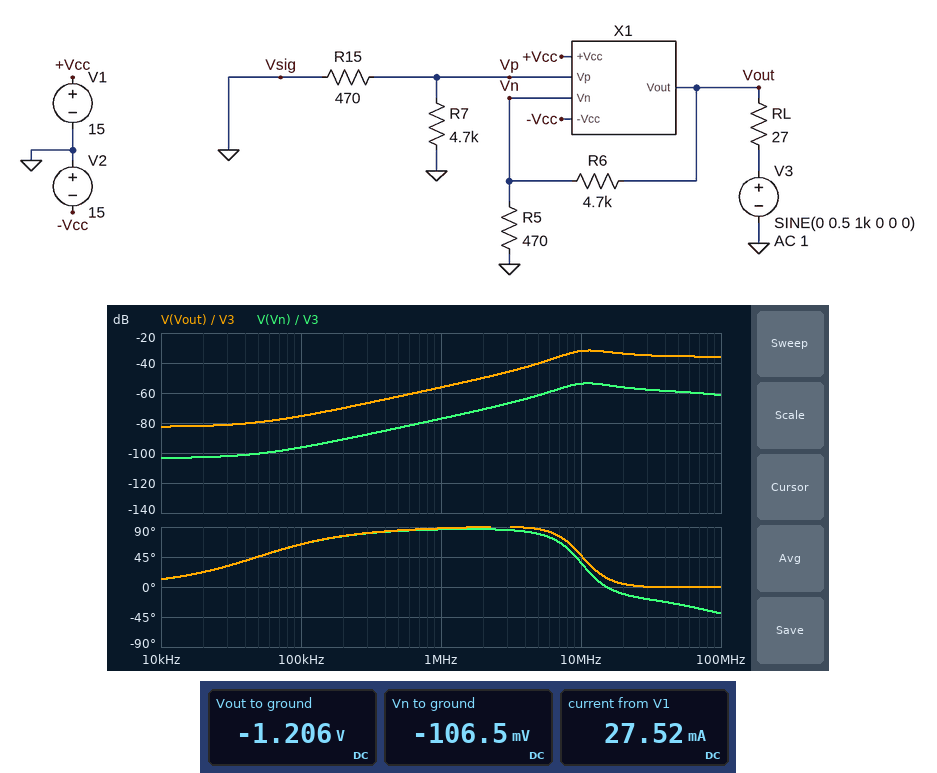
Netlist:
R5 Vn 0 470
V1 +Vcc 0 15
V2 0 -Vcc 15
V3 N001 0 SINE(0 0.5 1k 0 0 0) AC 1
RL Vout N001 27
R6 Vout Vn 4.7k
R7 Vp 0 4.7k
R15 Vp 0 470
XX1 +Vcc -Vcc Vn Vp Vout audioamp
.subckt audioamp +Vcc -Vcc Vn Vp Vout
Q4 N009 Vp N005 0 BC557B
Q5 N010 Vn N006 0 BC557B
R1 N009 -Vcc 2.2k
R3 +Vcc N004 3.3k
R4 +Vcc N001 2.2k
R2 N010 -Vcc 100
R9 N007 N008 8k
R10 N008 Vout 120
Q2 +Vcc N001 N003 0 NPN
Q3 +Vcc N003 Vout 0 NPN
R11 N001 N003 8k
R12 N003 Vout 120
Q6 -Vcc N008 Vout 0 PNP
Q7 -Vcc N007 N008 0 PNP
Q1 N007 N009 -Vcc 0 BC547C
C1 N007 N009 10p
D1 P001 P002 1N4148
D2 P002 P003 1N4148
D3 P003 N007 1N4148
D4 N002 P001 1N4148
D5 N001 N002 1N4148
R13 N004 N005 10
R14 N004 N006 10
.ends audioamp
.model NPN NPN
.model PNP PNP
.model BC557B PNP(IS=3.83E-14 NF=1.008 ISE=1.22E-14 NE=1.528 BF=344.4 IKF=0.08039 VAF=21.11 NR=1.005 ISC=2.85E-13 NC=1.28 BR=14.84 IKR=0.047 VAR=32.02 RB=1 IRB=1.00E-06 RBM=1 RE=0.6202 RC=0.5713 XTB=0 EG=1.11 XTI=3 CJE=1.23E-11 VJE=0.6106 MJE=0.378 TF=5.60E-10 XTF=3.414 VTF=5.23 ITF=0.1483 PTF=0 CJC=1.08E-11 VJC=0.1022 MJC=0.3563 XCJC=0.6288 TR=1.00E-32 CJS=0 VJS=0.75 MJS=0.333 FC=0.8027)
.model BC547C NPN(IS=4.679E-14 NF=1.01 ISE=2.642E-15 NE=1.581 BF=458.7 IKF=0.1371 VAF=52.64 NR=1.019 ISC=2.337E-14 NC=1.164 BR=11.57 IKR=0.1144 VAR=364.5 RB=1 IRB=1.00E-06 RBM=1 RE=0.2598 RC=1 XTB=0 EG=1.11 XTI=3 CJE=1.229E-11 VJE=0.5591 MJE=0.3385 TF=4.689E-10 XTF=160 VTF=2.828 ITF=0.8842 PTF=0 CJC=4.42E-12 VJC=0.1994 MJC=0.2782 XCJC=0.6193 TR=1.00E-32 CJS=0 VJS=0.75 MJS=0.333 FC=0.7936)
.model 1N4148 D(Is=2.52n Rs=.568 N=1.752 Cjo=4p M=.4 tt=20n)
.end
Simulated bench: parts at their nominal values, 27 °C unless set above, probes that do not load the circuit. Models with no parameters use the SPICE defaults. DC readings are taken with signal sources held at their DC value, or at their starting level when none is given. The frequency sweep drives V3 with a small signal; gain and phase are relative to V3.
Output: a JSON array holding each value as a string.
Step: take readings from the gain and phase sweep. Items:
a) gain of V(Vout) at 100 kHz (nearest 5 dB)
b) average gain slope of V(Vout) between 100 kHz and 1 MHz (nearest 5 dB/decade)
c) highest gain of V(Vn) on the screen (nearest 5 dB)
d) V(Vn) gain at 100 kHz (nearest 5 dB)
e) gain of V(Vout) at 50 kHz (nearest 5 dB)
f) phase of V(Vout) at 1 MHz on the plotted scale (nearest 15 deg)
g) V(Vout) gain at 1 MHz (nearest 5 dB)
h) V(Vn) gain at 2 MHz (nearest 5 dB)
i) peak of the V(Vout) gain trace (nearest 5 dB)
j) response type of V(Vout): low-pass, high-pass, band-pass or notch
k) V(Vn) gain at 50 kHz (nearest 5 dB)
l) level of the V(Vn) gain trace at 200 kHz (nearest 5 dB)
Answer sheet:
["-75 dB", "20 dB/decade", "-55 dB", "-95 dB", "-80 dB", "90 deg", "-55 dB", "-70 dB", "-30 dB", "high-pass", "-100 dB", "-90 dB"]
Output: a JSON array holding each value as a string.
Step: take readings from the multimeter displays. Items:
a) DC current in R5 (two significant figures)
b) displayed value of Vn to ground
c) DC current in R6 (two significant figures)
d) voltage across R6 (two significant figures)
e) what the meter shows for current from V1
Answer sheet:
["230 µA", "-106.5 mV", "230 µA", "1.1 V", "27.52 mA"]
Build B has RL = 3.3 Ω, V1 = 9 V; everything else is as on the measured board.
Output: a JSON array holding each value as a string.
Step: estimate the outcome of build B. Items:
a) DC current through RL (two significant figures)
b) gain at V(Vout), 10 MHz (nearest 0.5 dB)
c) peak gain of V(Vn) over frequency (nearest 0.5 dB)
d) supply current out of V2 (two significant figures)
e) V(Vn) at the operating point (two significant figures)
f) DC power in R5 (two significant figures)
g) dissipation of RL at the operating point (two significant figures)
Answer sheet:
["250 mA", "-24.0 dB", "-46.0 dB", "260 mA", "-73 mV", "11 µW", "200 mW"]
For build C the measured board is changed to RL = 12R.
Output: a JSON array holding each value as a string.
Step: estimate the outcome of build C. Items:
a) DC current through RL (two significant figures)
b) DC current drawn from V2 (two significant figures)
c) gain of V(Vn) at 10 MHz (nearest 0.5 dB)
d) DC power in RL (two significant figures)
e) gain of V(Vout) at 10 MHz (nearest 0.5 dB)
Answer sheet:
["100 mA", "120 mA", "-51.0 dB", "120 mW", "-29.0 dB"]
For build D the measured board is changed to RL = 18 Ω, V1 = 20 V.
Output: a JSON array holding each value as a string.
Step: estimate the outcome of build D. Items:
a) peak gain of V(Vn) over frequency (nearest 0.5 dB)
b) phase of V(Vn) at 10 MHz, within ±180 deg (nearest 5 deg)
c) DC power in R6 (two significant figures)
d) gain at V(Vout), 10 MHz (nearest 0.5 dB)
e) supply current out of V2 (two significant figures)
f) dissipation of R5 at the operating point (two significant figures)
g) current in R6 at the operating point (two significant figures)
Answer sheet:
["-59.0 dB", "40 deg", "390 µW", "-37.5 dB", "160 mA", "36 µW", "290 µA"]
